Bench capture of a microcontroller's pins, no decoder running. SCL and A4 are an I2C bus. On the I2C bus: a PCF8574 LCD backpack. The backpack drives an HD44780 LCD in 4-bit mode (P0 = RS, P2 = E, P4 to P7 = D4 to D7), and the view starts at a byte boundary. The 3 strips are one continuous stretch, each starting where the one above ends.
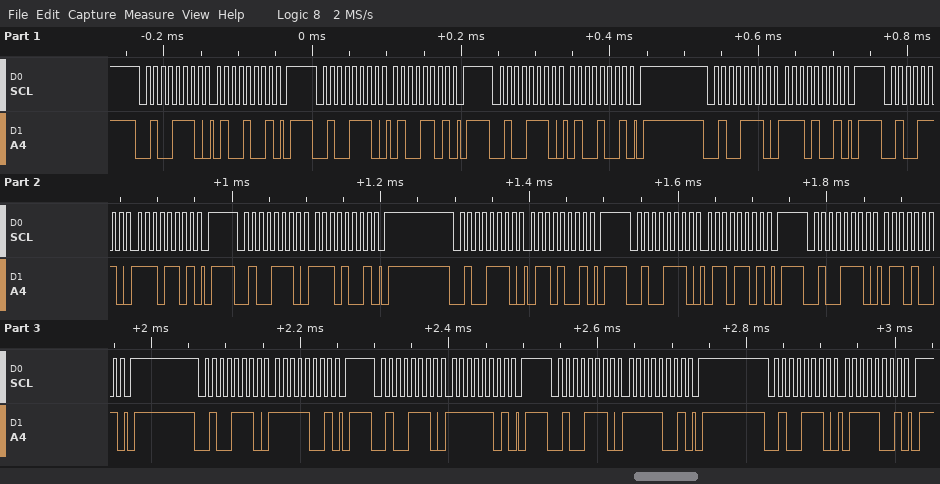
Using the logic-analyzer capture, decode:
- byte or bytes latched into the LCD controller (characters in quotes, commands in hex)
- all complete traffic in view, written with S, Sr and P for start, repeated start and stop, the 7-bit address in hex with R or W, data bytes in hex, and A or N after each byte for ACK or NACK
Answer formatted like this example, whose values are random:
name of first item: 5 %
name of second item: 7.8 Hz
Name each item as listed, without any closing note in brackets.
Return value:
byte or bytes latched into the LCD controller: 'N' 'o'
all complete traffic in view, written with S, Sr and P for start, repeated start and stop, the 7-bit address in hex with R or W, data bytes in hex, and A or N after each byte for ACK or NACK: S 27W A 49 A P S 27W A 4D A P S 27W A 49 A P S 27W A E9 A P S 27W A ED A P S 27W A E9 A P S 27W A 69 A P S 27W A 6D A P S 27W A 69 A P S 27W A F9 A P S 27W A FD A P S 27W A F9 A P S 27W A 79 A P
